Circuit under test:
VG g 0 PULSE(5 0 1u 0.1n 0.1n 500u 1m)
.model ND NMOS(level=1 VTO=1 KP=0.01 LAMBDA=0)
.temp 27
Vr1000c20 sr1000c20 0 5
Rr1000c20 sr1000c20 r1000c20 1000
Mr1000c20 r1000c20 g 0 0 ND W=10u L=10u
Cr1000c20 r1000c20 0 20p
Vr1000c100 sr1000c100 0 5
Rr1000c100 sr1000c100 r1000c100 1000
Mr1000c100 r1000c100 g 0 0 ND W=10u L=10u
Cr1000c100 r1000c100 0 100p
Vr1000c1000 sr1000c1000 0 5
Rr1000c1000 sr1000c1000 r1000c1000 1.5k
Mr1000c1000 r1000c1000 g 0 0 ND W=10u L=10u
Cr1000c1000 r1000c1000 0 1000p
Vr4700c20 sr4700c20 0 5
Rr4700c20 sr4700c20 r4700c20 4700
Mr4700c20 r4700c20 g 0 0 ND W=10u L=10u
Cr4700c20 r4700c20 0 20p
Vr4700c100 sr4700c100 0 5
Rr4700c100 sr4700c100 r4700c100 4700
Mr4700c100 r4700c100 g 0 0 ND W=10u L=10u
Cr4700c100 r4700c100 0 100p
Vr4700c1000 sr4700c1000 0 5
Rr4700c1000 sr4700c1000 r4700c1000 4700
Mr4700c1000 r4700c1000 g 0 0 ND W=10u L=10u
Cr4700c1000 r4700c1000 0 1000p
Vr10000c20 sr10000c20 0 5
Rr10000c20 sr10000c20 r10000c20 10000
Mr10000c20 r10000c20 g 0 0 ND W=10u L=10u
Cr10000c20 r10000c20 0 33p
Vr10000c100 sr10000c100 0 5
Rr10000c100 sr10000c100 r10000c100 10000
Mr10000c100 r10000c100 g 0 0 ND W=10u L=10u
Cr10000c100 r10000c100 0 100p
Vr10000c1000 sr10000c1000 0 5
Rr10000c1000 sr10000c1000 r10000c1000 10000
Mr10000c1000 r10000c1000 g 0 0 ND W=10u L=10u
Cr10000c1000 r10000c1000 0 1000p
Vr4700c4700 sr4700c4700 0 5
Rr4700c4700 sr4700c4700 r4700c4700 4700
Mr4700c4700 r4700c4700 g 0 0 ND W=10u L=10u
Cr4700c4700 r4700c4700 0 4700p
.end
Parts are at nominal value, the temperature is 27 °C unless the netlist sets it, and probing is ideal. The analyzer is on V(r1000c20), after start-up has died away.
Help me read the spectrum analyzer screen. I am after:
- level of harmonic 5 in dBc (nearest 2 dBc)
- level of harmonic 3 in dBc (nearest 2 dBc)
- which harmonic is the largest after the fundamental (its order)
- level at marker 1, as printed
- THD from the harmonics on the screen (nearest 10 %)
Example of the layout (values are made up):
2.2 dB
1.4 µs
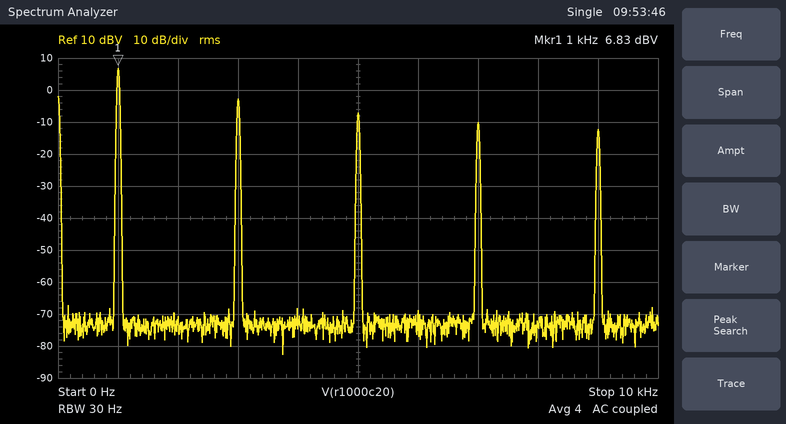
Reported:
-14 dBc
-10 dBc
3
6.83 dBV
40 %
